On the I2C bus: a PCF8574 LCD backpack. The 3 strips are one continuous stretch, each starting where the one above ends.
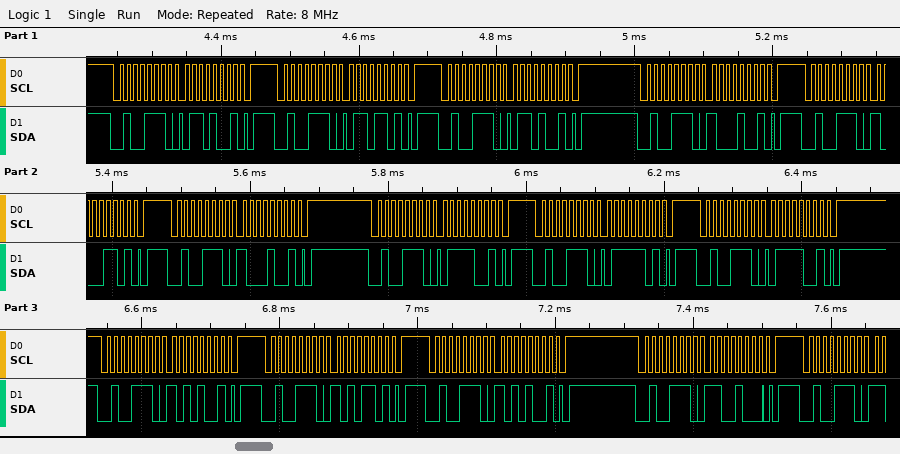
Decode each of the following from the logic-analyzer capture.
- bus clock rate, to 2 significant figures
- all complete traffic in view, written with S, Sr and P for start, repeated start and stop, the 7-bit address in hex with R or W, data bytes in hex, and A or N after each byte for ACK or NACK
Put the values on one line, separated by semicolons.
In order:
100 kHz; S 27W A 69 A P S 27W A 6D A P S 27W A 69 A P S 27W A 89 A P S 27W A 8D A P S 27W A 89 A P S 27W A 79 A P S 27W A 7D A P S 27W A 79 A P S 27W A A9 A P S 27W A AD A P S 27W A A9 A P S 27W A C8 A P S 27W A
